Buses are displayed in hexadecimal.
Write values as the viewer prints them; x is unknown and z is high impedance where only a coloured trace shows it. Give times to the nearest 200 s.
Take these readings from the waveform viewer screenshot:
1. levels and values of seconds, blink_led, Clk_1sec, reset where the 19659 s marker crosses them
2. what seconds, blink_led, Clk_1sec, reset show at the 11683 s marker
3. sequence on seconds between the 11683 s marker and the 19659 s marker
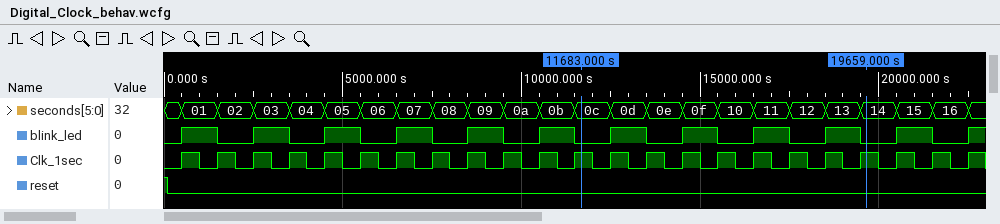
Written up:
seconds=14, blink_led=0, Clk_1sec=1, reset=0
seconds=0c, blink_led=0, Clk_1sec=1, reset=0
0c, 0d, 0e, 0f, 10, 11, 12, 13, 14
